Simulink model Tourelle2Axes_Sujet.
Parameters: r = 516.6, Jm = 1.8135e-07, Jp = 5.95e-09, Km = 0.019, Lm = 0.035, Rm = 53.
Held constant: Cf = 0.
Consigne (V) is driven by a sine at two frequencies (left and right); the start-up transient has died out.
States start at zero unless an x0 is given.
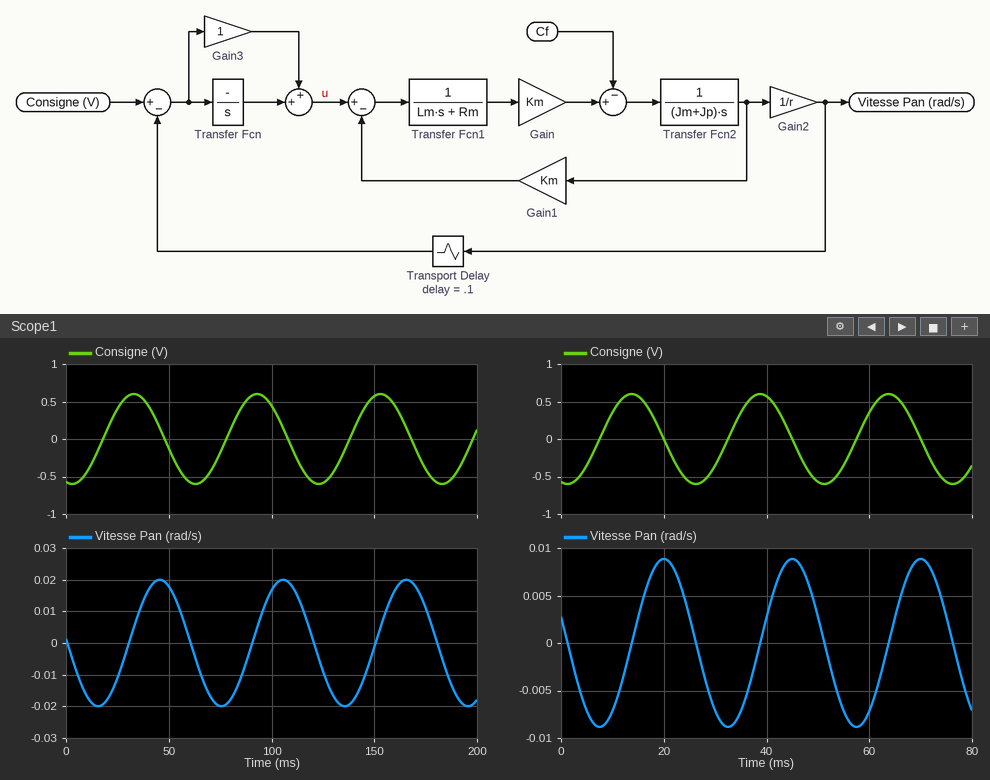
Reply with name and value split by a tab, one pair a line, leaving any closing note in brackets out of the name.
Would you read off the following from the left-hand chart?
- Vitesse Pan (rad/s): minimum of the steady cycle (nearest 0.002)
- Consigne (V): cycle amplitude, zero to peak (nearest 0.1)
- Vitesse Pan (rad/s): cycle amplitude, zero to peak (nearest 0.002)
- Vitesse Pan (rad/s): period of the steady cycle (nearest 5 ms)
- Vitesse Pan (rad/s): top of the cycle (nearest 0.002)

Vitesse Pan (rad/s): minimum of the steady cycle	-0.020
Consigne (V): cycle amplitude, zero to peak	0.6
Vitesse Pan (rad/s): cycle amplitude, zero to peak	0.020
Vitesse Pan (rad/s): period of the steady cycle	60 ms
Vitesse Pan (rad/s): top of the cycle	0.020
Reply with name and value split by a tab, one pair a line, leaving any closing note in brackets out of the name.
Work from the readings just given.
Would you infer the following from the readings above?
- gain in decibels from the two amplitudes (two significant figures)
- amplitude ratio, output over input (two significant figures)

gain in decibels from the two amplitudes	-30 dB
amplitude ratio, output over input	0.033
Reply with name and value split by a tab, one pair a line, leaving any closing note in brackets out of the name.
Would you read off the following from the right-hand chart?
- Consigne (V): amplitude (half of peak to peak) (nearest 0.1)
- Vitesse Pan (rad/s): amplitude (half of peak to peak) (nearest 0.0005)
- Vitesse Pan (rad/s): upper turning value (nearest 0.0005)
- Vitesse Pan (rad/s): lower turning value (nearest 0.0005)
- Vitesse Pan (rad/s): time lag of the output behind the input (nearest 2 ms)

Consigne (V): amplitude (half of peak to peak)	0.6
Vitesse Pan (rad/s): amplitude (half of peak to peak)	0.0090
Vitesse Pan (rad/s): upper turning value	0.0090
Vitesse Pan (rad/s): lower turning value	-0.0090
Vitesse Pan (rad/s): time lag of the output behind the input	6 ms
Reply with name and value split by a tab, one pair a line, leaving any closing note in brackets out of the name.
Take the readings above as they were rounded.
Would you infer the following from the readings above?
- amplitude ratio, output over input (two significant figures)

amplitude ratio, output over input	0.015
